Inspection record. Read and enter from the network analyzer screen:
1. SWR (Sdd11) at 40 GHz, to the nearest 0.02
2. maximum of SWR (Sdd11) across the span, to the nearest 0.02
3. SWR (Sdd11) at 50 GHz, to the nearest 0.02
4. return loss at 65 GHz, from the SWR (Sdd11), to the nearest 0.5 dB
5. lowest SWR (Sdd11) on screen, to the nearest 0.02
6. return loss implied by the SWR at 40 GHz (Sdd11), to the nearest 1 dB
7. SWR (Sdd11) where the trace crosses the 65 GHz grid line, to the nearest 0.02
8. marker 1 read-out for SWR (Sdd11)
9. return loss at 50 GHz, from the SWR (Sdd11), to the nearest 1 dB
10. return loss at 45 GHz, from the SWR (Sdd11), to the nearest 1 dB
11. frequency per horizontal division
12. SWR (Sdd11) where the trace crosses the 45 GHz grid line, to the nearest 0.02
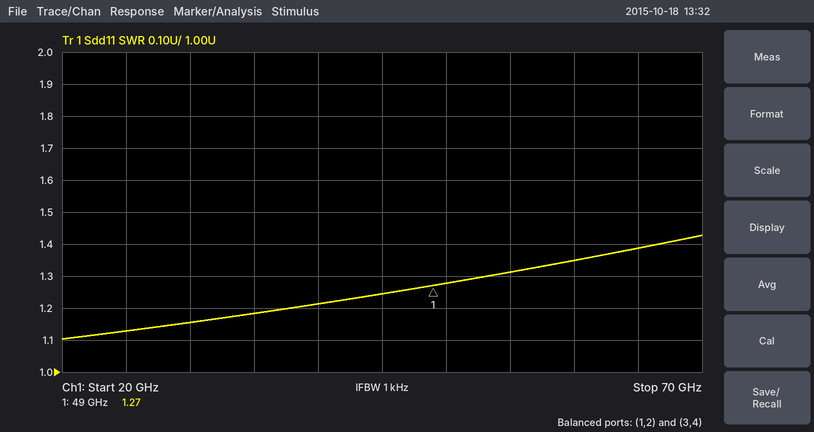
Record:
1.22
1.42
1.28
16.0 dB
1.10
20 dB
1.38
1.27
18 dB
19 dB
5 GHz
1.24
